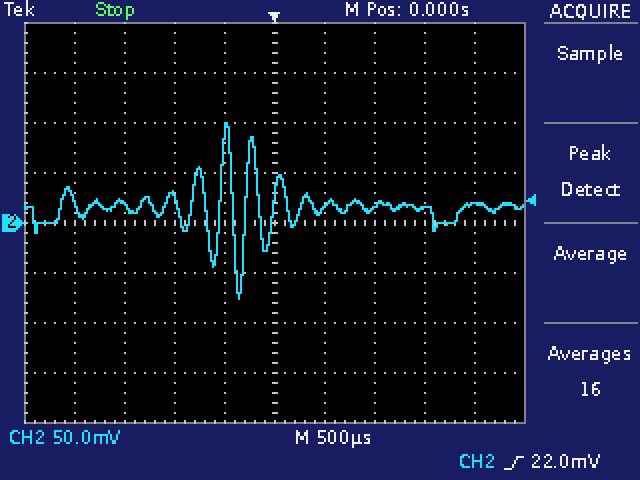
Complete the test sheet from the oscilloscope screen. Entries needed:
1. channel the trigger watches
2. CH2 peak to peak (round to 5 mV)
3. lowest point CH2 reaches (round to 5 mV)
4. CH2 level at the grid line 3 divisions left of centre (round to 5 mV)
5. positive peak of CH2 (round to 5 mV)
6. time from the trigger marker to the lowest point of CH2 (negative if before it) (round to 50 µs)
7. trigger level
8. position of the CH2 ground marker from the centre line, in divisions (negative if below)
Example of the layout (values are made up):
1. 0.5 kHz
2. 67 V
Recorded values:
1. CH2
2. 175 mV
3. -75 mV
4. 20 mV
5. 100 mV
6. -350 µs
7. 22.0 mV
8. 0.0 div
